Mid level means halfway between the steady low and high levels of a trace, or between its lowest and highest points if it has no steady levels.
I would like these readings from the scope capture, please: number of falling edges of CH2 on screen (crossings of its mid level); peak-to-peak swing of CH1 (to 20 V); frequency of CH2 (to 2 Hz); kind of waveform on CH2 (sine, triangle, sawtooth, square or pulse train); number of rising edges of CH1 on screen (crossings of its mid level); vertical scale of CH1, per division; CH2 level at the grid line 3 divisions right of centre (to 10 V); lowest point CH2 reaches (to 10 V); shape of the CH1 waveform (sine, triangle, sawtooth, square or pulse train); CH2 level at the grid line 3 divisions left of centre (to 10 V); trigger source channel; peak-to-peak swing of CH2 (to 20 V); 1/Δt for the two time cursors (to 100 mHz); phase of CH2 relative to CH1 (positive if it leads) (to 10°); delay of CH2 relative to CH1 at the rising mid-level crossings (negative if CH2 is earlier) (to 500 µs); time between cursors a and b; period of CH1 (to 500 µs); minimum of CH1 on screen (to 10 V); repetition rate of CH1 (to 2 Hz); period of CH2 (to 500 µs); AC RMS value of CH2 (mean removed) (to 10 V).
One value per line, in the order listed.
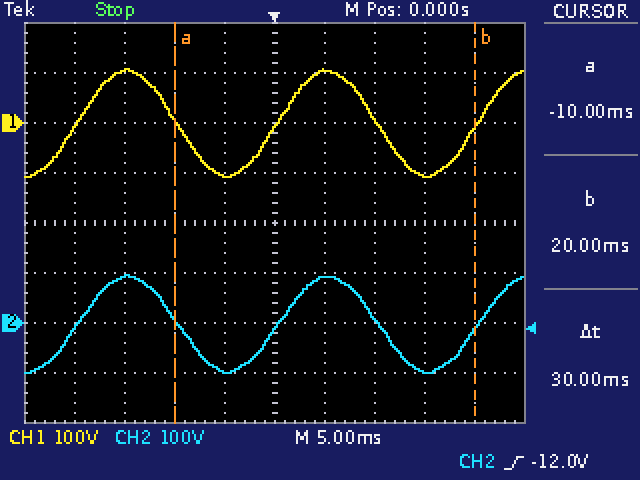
2
220 V
50 Hz
sine
3
100 V
-100 V
-100 V
sine
90 V
CH2
200 V
33.3 Hz
0°
0.0 ms
30 ms
20.0 ms
-110 V
50 Hz
20.0 ms
70 V
